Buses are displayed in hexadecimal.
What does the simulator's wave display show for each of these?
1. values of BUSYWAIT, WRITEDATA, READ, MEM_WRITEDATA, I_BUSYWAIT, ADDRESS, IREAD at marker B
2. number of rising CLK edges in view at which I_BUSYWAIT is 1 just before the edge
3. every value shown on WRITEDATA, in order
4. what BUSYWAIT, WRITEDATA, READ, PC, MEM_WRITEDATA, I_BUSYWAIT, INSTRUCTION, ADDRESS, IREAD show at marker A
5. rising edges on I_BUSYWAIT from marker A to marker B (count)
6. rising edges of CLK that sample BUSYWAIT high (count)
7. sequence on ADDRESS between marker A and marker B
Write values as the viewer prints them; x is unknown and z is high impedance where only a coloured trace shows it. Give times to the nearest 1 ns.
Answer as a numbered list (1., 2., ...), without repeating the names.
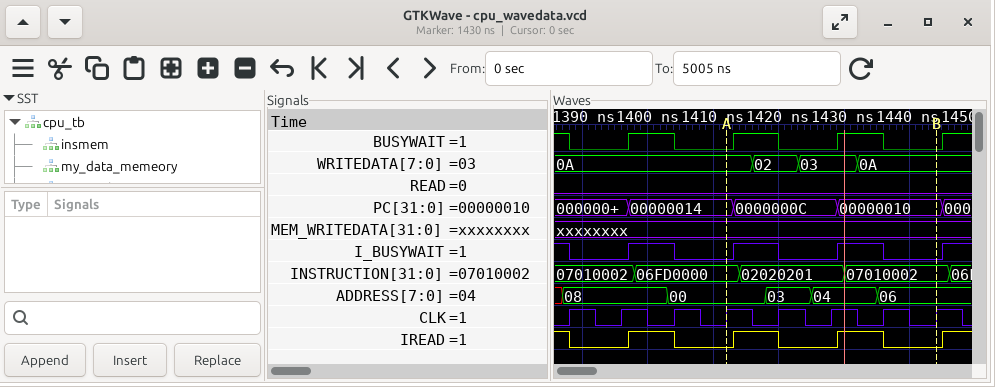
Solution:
1. BUSYWAIT=0, WRITEDATA=0A, READ=0, MEM_WRITEDATA=xxxxxxxx, I_BUSYWAIT=0, ADDRESS=06, IREAD=0
2. 4
3. 0A, 02, 03, 0A
4. BUSYWAIT=0, WRITEDATA=0A, READ=0, PC=00000014, MEM_WRITEDATA=xxxxxxxx, I_BUSYWAIT=0, INSTRUCTION=06FD0000, ADDRESS=00, IREAD=0
5. 2
6. 4
7. 00, 03, 04, 06
